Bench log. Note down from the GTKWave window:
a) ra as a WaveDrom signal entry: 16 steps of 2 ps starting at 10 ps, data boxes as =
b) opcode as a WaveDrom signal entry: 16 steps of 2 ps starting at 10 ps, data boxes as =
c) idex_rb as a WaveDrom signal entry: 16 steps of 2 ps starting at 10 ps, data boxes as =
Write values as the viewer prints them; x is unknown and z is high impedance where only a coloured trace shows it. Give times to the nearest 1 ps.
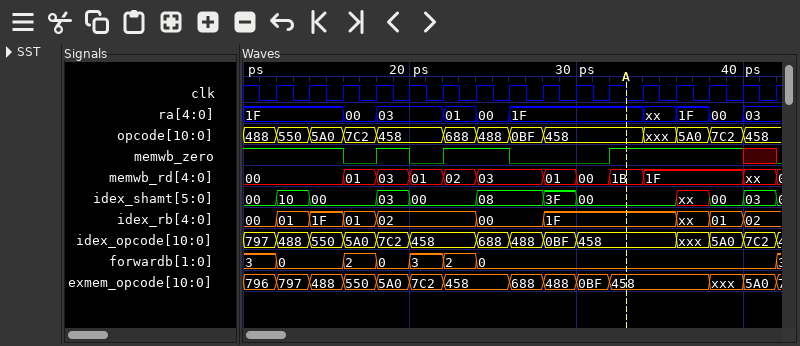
{name: 'ra', wave: '=..==.===...x===', data: '1F 00 03 01 00 1F 1F 00 03'}
{name: 'opcode', wave: '=====.====..x===', data: '488 550 5A0 7C2 458 688 488 0BF 458 5A0 7C2 458'}
{name: 'idex_rb', wave: '=====..=.=...x==', data: '00 01 1F 01 02 00 1F 01 02'}
